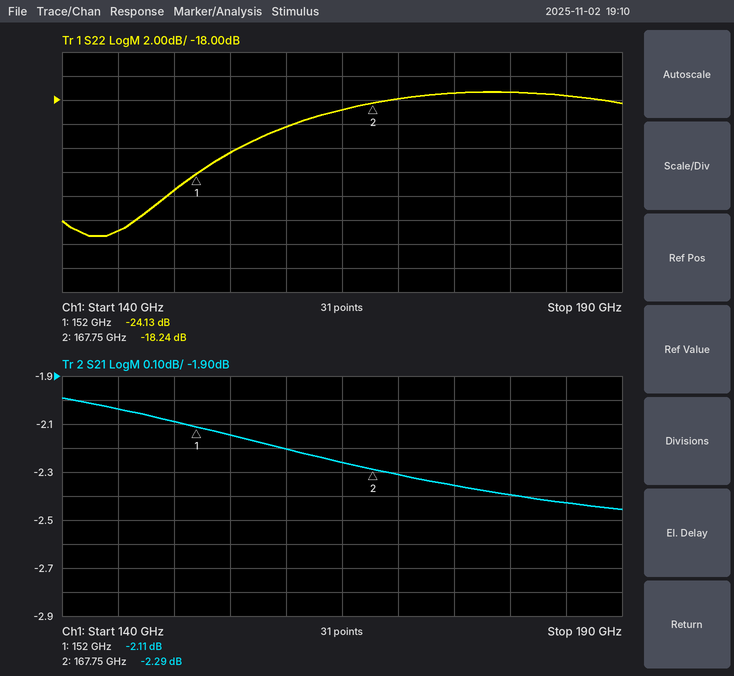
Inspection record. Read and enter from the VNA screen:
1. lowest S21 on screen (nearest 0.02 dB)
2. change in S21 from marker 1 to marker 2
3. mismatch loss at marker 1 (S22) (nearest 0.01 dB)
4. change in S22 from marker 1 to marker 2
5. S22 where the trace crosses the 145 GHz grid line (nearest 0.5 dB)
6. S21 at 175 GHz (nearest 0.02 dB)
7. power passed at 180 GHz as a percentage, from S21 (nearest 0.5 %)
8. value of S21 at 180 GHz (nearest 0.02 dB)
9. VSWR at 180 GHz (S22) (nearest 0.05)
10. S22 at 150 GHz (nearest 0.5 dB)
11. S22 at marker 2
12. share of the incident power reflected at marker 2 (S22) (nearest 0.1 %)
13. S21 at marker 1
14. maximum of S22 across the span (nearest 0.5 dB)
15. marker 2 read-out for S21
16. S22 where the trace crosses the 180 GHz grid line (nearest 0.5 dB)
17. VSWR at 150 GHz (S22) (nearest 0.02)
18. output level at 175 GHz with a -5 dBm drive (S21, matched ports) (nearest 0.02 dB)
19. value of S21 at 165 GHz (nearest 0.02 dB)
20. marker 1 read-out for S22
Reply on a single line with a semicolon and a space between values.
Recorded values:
-2.46 dB; -0.18 dB; 0.02 dB; 5.89 dB; -29.0 dB; -2.36 dB; 57.5 %; -2.40 dB; 1.30; -25.5 dB; -18.24 dB; 1.5 %; -2.11 dB; -17.5 dB; -2.29 dB; -17.5 dB; 1.12; -7.36 dBm; -2.26 dB; -24.13 dB
